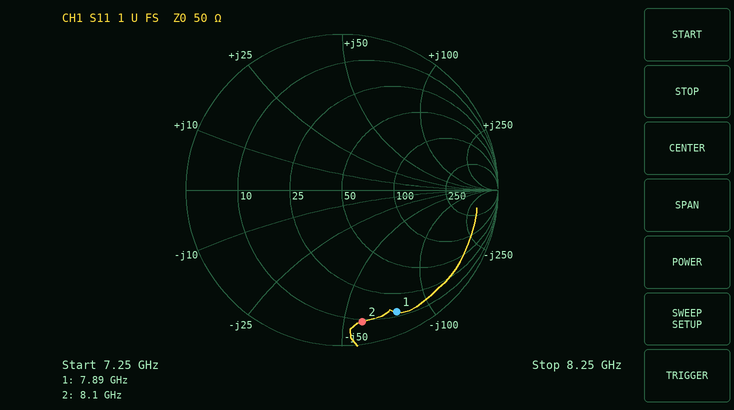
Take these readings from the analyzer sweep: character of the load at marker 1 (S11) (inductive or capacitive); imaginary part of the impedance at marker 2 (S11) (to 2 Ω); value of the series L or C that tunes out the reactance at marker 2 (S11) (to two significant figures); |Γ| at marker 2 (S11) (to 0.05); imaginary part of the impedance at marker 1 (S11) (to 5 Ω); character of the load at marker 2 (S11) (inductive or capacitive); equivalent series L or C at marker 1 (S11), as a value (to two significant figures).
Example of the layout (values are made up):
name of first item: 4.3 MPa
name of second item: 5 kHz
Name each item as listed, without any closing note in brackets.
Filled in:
character of the load at marker 1 (S11): capacitive
imaginary part of the impedance at marker 2 (S11): -58 Ω
value of the series L or C that tunes out the reactance at marker 2 (S11): 1.1 nH
|Γ| at marker 2 (S11): 0.85
imaginary part of the impedance at marker 1 (S11): -75 Ω
character of the load at marker 2 (S11): capacitive
equivalent series L or C at marker 1 (S11), as a value: 270 fF
